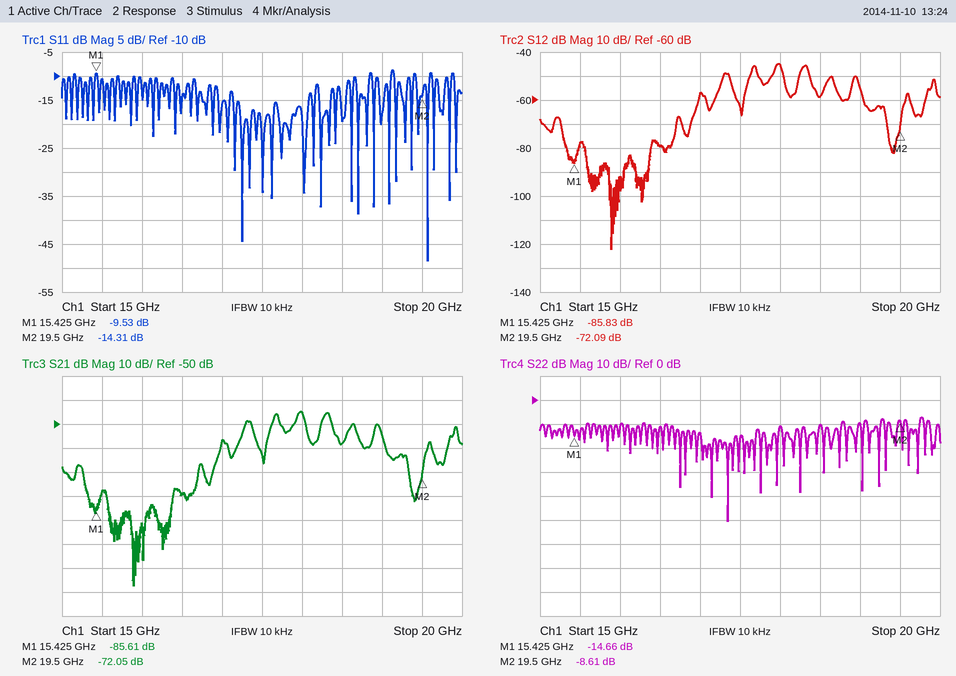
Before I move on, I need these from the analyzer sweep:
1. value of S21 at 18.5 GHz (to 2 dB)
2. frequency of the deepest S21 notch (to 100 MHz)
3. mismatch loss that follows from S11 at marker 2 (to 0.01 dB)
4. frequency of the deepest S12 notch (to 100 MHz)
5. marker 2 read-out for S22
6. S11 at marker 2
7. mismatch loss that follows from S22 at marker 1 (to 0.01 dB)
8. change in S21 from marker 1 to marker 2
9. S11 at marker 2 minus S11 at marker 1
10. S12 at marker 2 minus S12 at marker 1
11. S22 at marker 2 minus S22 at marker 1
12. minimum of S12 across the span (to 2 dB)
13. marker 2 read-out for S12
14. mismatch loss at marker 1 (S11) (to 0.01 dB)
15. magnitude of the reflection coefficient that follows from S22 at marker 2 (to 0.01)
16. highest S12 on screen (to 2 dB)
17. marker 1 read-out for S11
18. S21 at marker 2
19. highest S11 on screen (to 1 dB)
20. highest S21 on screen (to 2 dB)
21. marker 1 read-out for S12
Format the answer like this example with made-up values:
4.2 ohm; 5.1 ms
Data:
-58 dB; 15.9 GHz; 0.16 dB; 15.9 GHz; -8.61 dB; -14.31 dB; 0.15 dB; 13.56 dB; -4.78 dB; 13.74 dB; 6.05 dB; -122 dB; -72.09 dB; 0.51 dB; 0.37; -44 dB; -9.53 dB; -72.05 dB; -9 dB; -44 dB; -85.83 dB
